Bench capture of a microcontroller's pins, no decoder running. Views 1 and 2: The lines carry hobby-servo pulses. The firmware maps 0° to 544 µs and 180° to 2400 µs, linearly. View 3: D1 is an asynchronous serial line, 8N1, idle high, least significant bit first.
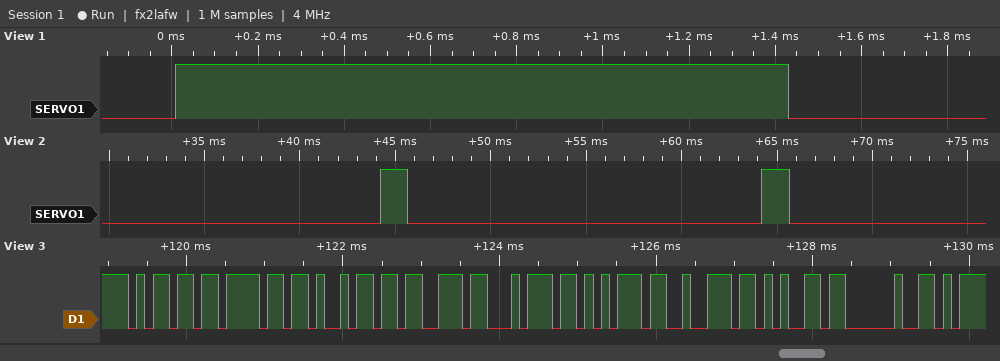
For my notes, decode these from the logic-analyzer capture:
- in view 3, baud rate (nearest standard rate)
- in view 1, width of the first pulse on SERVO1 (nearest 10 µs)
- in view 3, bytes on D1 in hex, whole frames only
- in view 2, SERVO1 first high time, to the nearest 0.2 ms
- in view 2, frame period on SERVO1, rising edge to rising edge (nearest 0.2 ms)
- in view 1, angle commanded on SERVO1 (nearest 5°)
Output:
9600 baud
1420 µs
6D 6F 69 73 74 75 72 65 20
1.4 ms
20.0 ms
85°
